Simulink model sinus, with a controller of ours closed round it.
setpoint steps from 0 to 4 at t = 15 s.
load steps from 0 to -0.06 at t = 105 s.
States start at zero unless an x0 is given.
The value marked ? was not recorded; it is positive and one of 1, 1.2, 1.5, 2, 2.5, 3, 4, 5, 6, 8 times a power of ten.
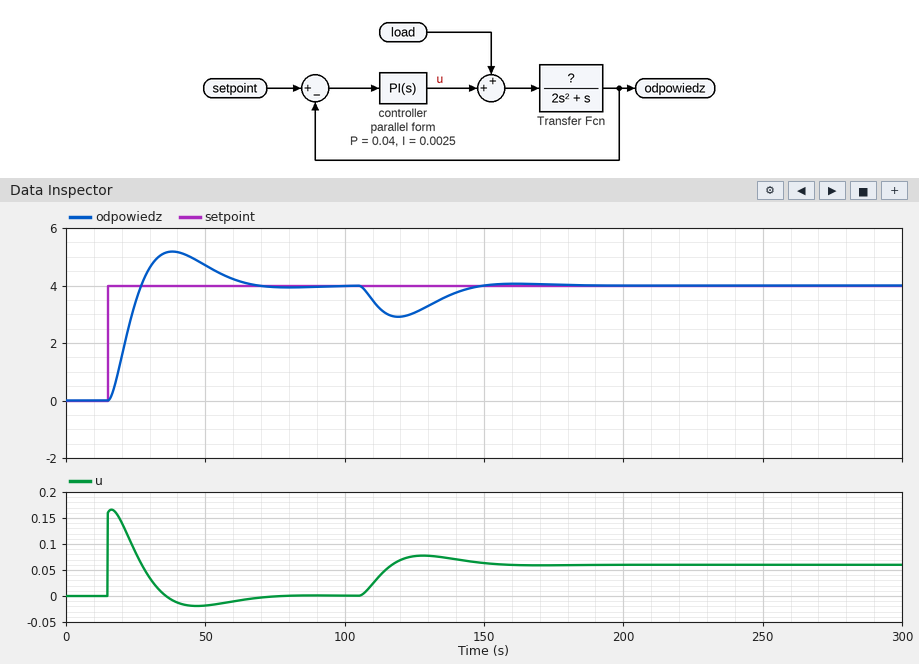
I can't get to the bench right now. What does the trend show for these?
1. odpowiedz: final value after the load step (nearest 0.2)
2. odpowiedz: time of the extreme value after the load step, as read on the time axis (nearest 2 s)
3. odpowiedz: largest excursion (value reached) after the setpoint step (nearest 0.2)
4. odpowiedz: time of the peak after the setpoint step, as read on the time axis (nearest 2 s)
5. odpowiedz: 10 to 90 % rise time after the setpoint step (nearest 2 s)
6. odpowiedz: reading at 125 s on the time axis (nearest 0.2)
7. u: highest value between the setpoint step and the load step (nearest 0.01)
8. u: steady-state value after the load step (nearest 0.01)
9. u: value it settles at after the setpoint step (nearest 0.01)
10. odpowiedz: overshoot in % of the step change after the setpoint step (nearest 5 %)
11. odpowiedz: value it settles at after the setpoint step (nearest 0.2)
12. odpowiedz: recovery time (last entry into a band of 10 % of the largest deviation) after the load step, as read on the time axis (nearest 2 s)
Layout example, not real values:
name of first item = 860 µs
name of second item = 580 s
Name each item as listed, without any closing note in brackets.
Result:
odpowiedz: final value after the load step = 4.0
odpowiedz: time of the extreme value after the load step, as read on the time axis = 120 s
odpowiedz: largest excursion (value reached) after the setpoint step = 5.2
odpowiedz: time of the peak after the setpoint step, as read on the time axis = 38 s
odpowiedz: 10 to 90 % rise time after the setpoint step = 8 s
odpowiedz: reading at 125 s on the time axis = 3.0
u: highest value between the setpoint step and the load step = 0.17
u: steady-state value after the load step = 0.06
u: value it settles at after the setpoint step = 0.00
odpowiedz: overshoot in % of the step change after the setpoint step = 30 %
odpowiedz: value it settles at after the setpoint step = 4.0
odpowiedz: recovery time (last entry into a band of 10 % of the largest deviation) after the load step, as read on the time axis = 144 s
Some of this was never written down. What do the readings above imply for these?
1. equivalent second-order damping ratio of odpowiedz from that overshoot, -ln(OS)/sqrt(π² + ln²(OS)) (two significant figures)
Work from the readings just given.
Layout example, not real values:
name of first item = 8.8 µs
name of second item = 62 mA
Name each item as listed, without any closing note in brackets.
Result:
equivalent second-order damping ratio of odpowiedz from that overshoot, -ln(OS)/sqrt(π² + ln²(OS)) = 0.36
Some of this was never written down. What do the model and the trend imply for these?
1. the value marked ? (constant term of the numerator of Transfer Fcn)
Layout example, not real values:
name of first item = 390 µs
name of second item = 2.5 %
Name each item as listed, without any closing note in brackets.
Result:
the value marked ? = 3
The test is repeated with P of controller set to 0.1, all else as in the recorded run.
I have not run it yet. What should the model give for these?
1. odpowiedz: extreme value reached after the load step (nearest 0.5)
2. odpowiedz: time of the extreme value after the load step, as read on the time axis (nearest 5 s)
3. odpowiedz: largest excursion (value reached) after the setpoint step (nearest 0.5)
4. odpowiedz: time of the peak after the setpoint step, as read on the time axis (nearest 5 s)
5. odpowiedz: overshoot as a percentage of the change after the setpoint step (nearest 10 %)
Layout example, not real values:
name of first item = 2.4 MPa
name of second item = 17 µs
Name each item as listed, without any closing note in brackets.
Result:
odpowiedz: extreme value reached after the load step = 3.5
odpowiedz: time of the extreme value after the load step, as read on the time axis = 115 s
odpowiedz: largest excursion (value reached) after the setpoint step = 4.5
odpowiedz: time of the peak after the setpoint step, as read on the time axis = 25 s
odpowiedz: overshoot as a percentage of the change after the setpoint step = 20 %
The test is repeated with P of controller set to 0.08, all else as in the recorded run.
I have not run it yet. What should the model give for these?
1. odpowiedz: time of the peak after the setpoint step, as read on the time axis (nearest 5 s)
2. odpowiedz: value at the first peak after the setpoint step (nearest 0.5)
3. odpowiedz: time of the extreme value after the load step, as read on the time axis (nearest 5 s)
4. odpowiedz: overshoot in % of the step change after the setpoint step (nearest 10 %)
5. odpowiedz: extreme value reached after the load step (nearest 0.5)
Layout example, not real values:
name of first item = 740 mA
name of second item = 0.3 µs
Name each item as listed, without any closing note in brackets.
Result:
odpowiedz: time of the peak after the setpoint step, as read on the time axis = 30 s
odpowiedz: value at the first peak after the setpoint step = 4.5
odpowiedz: time of the extreme value after the load step, as read on the time axis = 115 s
odpowiedz: overshoot in % of the step change after the setpoint step = 20 %
odpowiedz: extreme value reached after the load step = 3.5
